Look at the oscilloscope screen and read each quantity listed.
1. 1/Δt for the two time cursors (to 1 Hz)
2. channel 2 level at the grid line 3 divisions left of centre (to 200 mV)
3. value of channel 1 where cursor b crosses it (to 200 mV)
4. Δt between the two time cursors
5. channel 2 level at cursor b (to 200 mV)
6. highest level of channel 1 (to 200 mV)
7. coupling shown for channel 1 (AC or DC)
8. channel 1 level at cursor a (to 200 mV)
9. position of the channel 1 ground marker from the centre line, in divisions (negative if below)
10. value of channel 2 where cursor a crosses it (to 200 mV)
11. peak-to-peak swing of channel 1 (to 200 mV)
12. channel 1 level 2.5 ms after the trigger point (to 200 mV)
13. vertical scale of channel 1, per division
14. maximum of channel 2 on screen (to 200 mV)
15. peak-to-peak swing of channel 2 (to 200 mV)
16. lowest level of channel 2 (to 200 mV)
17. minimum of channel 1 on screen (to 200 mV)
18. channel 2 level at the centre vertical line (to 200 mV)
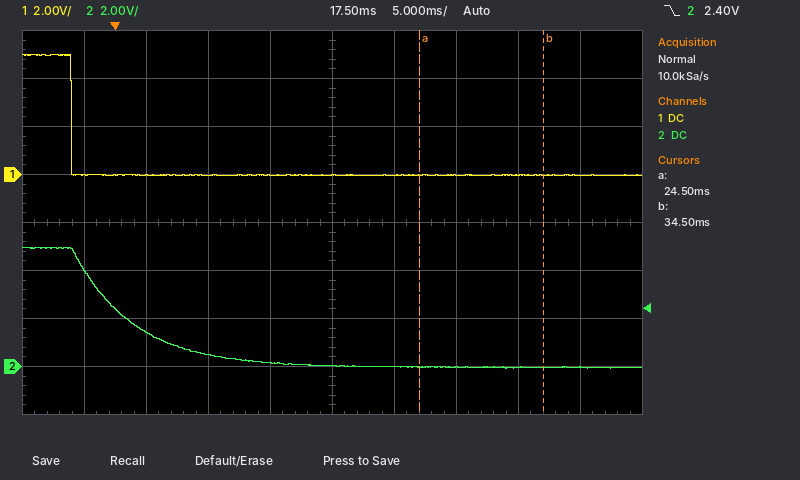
100 Hz
1.4 V
0.0 V
10.0 ms
0.0 V
5.0 V
DC
0.0 V
+1.0 div
0.0 V
5.0 V
0.0 V
2 V
5.0 V
5.0 V
0.0 V
0.0 V
0.0 V
